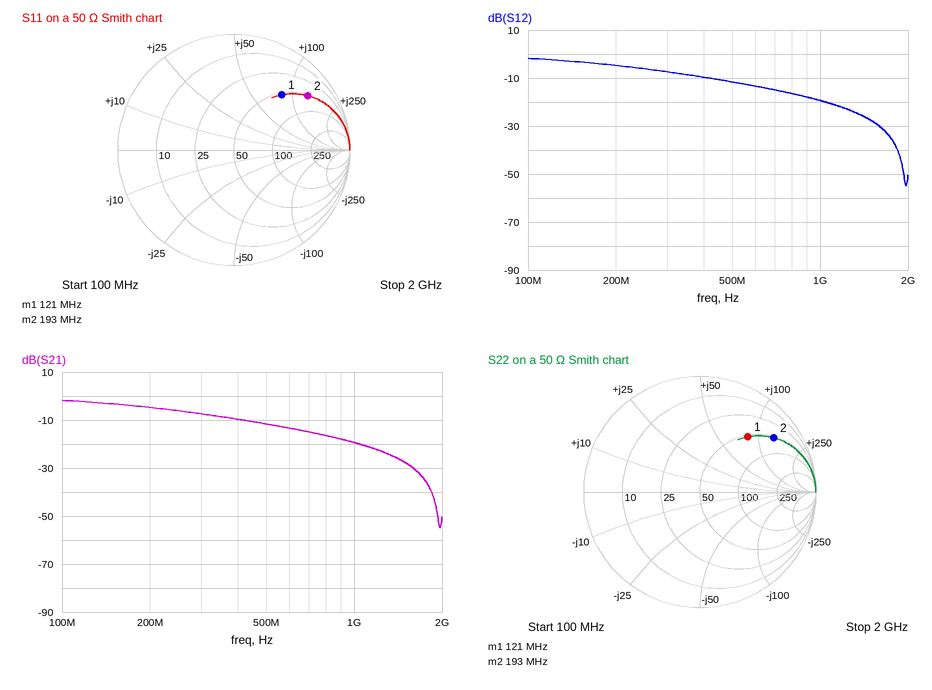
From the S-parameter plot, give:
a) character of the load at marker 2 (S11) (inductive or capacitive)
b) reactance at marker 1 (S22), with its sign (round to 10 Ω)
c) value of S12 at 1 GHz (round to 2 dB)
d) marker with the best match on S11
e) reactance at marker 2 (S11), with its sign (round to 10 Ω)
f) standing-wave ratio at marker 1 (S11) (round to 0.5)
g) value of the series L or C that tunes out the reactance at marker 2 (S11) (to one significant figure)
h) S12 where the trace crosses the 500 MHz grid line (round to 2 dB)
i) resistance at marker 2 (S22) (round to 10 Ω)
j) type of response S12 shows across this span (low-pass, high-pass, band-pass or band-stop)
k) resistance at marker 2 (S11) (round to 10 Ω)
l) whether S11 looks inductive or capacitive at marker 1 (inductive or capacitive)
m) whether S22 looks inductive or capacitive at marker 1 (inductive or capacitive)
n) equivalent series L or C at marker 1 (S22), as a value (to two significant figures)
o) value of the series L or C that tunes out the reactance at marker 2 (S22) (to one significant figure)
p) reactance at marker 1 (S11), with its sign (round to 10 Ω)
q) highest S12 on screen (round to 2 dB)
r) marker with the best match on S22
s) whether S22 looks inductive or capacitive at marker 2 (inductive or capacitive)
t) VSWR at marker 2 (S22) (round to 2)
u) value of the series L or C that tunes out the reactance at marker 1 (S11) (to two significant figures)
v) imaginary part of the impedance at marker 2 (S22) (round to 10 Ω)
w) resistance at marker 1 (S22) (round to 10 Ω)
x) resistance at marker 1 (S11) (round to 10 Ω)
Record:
inductive
+80 Ω
-20 dB
marker 1
+130 Ω
4.5
6 pF
-12 dB
50 Ω
low-pass
50 Ω
inductive
inductive
110 nH
6 pF
+80 Ω
-2 dB
marker 1
inductive
8
16 pF
+130 Ω
50 Ω
50 Ω
